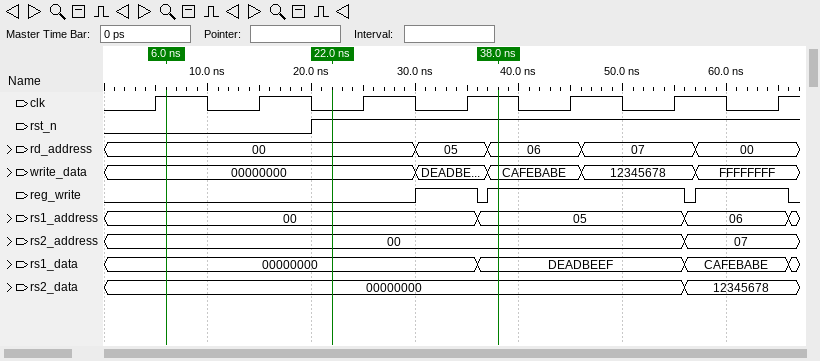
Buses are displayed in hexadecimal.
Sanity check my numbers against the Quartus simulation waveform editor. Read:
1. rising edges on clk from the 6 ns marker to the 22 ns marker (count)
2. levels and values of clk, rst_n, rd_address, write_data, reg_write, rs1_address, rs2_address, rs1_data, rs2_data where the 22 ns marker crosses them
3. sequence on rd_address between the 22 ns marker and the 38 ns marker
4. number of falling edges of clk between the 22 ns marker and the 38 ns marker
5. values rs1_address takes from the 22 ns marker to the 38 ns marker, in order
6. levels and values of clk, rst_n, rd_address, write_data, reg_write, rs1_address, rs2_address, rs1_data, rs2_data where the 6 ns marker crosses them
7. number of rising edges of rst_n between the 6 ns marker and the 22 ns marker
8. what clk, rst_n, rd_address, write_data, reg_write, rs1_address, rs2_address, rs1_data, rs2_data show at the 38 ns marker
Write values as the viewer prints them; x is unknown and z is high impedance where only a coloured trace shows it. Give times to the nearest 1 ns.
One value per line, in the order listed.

1
clk=0, rst_n=1, rd_address=00, write_data=00000000, reg_write=0, rs1_address=00, rs2_address=00, rs1_data=00000000, rs2_data=00000000
00, 05, 06
1
00, 05
clk=1, rst_n=0, rd_address=00, write_data=00000000, reg_write=0, rs1_address=00, rs2_address=00, rs1_data=00000000, rs2_data=00000000
1
clk=1, rst_n=1, rd_address=06, write_data=CAFEBABE, reg_write=1, rs1_address=05, rs2_address=00, rs1_data=DEADBEEF, rs2_data=00000000
